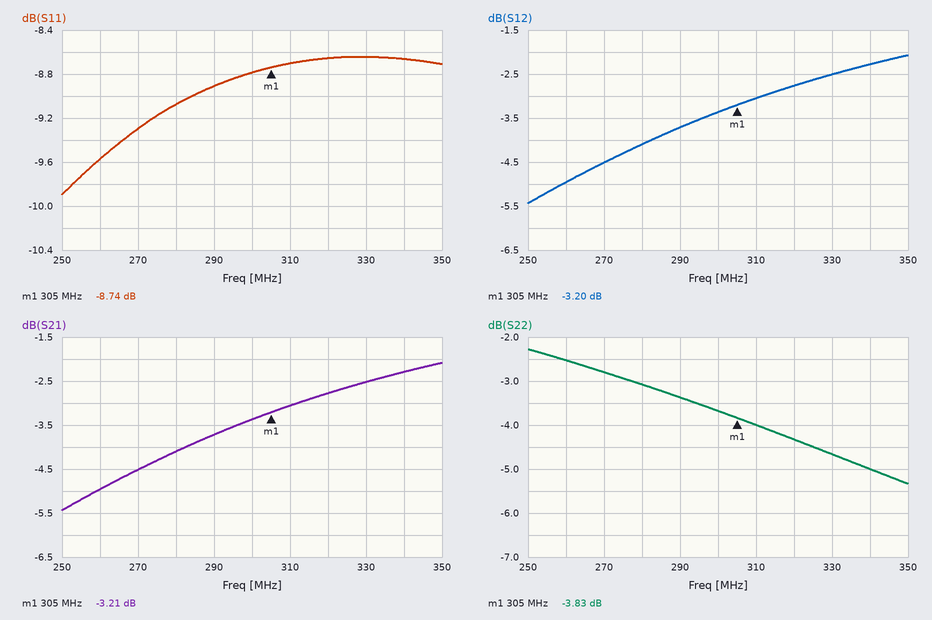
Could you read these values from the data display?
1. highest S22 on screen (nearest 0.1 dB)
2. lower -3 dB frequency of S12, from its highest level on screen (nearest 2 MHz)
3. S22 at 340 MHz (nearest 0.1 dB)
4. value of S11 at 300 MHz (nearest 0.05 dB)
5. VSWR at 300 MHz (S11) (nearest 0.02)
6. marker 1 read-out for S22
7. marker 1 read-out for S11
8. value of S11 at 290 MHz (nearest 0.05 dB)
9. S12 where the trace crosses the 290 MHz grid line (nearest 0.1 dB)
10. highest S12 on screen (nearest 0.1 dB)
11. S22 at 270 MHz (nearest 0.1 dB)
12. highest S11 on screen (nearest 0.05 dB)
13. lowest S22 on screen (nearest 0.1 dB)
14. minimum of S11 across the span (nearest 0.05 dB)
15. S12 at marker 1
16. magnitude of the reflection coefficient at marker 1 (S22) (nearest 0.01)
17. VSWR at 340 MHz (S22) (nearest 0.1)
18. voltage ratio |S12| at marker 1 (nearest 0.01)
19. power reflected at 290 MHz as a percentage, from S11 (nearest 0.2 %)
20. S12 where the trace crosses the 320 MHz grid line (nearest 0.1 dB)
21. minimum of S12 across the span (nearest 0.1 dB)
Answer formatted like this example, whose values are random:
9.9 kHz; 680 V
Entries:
-2.3 dB; 258 MHz; -5.0 dB; -8.80 dB; 2.14; -3.83 dB; -8.74 dB; -8.90 dB; -3.7 dB; -2.1 dB; -2.8 dB; -8.65 dB; -5.3 dB; -9.90 dB; -3.20 dB; 0.64; 3.6; 0.69; 12.8 %; -2.8 dB; -5.4 dB
